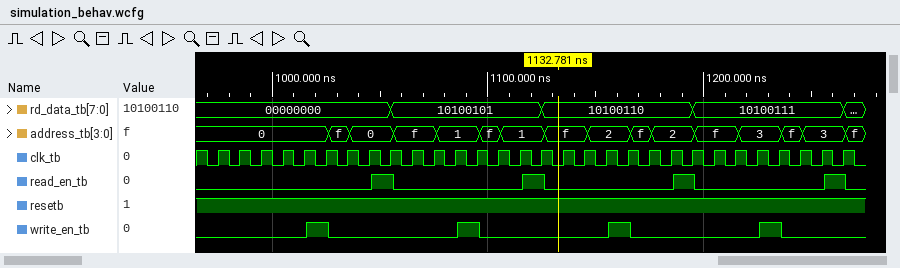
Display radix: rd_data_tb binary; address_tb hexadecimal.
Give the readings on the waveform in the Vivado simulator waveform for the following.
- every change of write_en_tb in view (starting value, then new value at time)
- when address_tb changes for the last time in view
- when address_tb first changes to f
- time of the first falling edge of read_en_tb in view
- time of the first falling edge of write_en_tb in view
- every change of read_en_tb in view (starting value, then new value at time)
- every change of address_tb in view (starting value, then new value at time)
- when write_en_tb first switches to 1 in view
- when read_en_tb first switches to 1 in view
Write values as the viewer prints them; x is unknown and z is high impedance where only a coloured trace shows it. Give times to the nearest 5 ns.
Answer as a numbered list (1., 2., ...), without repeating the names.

1. 0, 1 at 1015 ns, 0 at 1025 ns, 1 at 1085 ns, 0 at 1095 ns, 1 at 1155 ns, 0 at 1165 ns, 1 at 1225 ns, 0 at 1235 ns
2. 1265 ns
3. 1025 ns
4. 1055 ns
5. 1025 ns
6. 0, 1 at 1045 ns, 0 at 1055 ns, 1 at 1115 ns, 0 at 1125 ns, 1 at 1185 ns, 0 at 1195 ns, 1 at 1255 ns, 0 at 1265 ns
7. 0, f at 1025 ns, 0 at 1035 ns, f at 1055 ns, 1 at 1075 ns, f at 1095 ns, 1 at 1105 ns, f at 1125 ns, 2 at 1145 ns, f at 1165 ns, 2 at 1175 ns, f at 1195 ns, 3 at 1215 ns, f at 1235 ns, 3 at 1245 ns, f at 1265 ns
8. 1015 ns
9. 1045 ns
